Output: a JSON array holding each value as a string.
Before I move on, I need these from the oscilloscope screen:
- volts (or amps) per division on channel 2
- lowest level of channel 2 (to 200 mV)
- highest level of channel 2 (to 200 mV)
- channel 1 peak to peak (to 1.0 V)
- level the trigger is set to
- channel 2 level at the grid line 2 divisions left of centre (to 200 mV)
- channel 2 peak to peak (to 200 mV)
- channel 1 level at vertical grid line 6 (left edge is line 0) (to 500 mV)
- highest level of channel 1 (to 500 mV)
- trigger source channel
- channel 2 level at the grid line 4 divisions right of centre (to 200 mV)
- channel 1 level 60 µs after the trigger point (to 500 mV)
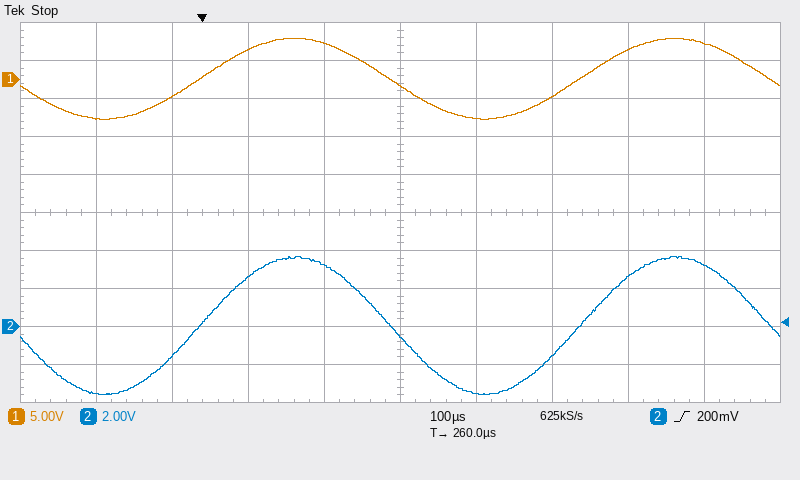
["2 V", "-3.6 V", "3.6 V", "11.0 V", "200 mV", "2.6 V", "7.2 V", "-5.0 V", "5.5 V", "channel 2", "3.2 V", "4.0 V"]
